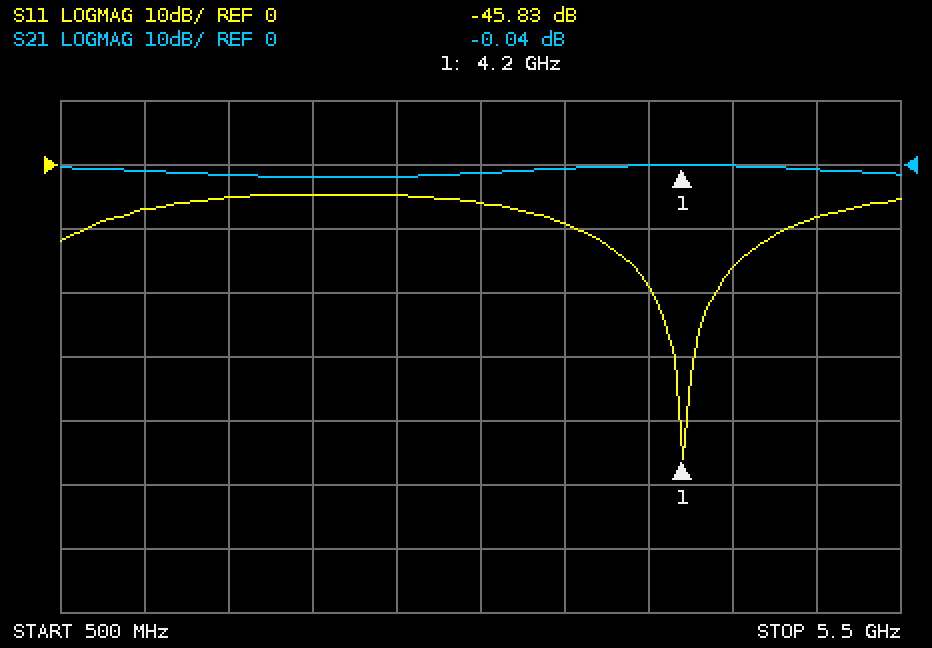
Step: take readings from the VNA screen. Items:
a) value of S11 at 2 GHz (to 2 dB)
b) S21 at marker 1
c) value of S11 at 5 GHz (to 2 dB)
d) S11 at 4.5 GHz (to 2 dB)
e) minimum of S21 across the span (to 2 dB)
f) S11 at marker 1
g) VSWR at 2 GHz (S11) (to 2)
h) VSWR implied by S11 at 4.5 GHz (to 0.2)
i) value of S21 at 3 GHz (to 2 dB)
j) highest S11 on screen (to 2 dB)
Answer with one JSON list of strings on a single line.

["-4 dB", "-0.04 dB", "-8 dB", "-16 dB", "-2 dB", "-45.83 dB", "4", "1.4", "-2 dB", "-4 dB"]
